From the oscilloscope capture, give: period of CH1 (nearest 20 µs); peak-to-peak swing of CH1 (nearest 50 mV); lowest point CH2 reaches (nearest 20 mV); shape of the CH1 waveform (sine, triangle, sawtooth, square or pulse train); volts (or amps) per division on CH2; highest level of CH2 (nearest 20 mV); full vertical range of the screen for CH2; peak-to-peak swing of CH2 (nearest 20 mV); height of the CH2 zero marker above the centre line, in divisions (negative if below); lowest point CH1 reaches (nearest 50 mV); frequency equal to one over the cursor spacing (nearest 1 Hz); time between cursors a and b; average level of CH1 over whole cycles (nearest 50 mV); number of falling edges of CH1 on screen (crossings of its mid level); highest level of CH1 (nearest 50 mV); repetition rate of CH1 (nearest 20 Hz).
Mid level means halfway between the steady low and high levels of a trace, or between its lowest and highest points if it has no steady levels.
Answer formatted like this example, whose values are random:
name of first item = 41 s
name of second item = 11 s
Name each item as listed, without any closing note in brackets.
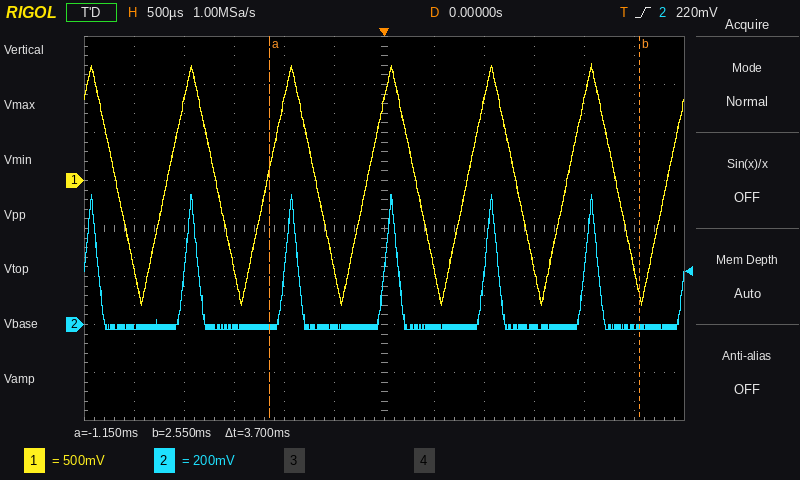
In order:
period of CH1 = 1.00 ms
peak-to-peak swing of CH1 = 2.50 V
lowest point CH2 reaches = -20 mV
shape of the CH1 waveform = triangle
volts (or amps) per division on CH2 = 200 mV
highest level of CH2 = 540 mV
full vertical range of the screen for CH2 = 1.6 V
peak-to-peak swing of CH2 = 560 mV
height of the CH2 zero marker above the centre line, in divisions = -2.0 div
lowest point CH1 reaches = -1.30 V
frequency equal to one over the cursor spacing = 270 Hz
time between cursors a and b = 3.7 ms
average level of CH1 over whole cycles = -50 mV
number of falling edges of CH1 on screen = 6
highest level of CH1 = 1.20 V
repetition rate of CH1 = 1.00 kHz
